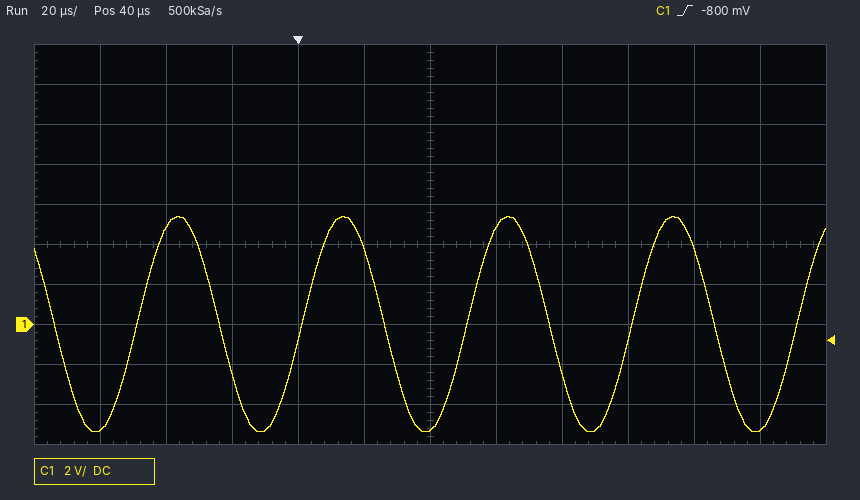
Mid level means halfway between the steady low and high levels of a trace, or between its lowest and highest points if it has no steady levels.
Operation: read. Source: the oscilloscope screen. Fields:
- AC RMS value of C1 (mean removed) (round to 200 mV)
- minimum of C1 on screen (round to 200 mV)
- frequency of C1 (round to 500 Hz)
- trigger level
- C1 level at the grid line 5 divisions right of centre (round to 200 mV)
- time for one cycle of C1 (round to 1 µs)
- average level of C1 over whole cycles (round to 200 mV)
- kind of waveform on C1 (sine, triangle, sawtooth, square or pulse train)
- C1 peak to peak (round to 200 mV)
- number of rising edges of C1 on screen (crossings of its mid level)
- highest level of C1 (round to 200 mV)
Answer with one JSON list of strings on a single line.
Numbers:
["3.8 V", "-5.4 V", "20.0 kHz", "-800 mV", "-5.2 V", "50 µs", "0.0 V", "sine", "10.8 V", "5", "5.4 V"]
